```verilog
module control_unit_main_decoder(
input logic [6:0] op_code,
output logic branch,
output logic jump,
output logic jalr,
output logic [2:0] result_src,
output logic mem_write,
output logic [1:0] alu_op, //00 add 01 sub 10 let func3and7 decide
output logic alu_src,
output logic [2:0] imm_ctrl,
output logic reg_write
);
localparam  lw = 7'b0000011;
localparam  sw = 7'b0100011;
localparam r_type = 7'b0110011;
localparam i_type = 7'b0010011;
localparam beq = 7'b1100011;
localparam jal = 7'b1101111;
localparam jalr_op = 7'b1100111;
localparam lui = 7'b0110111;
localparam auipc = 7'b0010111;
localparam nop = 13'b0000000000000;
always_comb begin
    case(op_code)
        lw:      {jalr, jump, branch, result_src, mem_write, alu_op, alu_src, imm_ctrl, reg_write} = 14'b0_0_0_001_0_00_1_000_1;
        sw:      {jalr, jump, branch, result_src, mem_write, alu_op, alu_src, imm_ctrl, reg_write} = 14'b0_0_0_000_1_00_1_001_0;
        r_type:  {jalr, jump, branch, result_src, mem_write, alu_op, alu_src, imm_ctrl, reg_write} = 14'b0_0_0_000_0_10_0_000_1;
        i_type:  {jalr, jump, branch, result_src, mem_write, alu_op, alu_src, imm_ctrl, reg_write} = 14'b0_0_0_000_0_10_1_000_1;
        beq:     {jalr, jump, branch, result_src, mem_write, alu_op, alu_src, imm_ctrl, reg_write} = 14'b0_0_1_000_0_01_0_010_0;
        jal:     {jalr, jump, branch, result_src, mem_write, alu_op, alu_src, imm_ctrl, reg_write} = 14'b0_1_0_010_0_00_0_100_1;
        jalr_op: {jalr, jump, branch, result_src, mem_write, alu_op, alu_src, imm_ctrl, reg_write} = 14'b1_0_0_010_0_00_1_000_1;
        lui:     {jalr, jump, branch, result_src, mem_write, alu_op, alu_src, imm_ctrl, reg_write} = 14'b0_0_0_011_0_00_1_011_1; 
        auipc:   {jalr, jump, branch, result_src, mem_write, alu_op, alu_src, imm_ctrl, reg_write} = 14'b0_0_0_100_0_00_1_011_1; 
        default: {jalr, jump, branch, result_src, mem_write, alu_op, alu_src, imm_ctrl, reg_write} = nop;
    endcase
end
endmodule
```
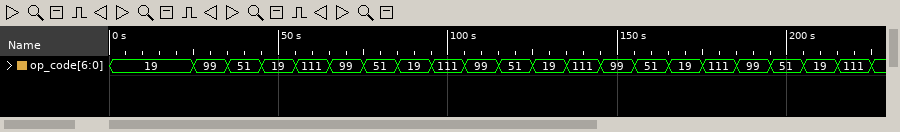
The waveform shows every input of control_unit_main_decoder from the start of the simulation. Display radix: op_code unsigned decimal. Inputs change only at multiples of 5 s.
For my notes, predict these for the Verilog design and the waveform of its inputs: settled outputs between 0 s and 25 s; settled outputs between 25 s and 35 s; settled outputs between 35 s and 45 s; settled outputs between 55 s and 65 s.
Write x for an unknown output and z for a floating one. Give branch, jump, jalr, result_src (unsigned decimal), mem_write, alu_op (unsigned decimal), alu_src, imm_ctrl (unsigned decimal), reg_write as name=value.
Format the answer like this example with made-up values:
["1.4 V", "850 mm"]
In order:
["branch=0, jump=0, jalr=0, result_src=0, mem_write=0, alu_op=2, alu_src=1, imm_ctrl=0, reg_write=1", "branch=1, jump=0, jalr=0, result_src=0, mem_write=0, alu_op=1, alu_src=0, imm_ctrl=2, reg_write=0", "branch=0, jump=0, jalr=0, result_src=0, mem_write=0, alu_op=2, alu_src=0, imm_ctrl=0, reg_write=1", "branch=0, jump=1, jalr=0, result_src=2, mem_write=0, alu_op=0, alu_src=0, imm_ctrl=4, reg_write=1"]
